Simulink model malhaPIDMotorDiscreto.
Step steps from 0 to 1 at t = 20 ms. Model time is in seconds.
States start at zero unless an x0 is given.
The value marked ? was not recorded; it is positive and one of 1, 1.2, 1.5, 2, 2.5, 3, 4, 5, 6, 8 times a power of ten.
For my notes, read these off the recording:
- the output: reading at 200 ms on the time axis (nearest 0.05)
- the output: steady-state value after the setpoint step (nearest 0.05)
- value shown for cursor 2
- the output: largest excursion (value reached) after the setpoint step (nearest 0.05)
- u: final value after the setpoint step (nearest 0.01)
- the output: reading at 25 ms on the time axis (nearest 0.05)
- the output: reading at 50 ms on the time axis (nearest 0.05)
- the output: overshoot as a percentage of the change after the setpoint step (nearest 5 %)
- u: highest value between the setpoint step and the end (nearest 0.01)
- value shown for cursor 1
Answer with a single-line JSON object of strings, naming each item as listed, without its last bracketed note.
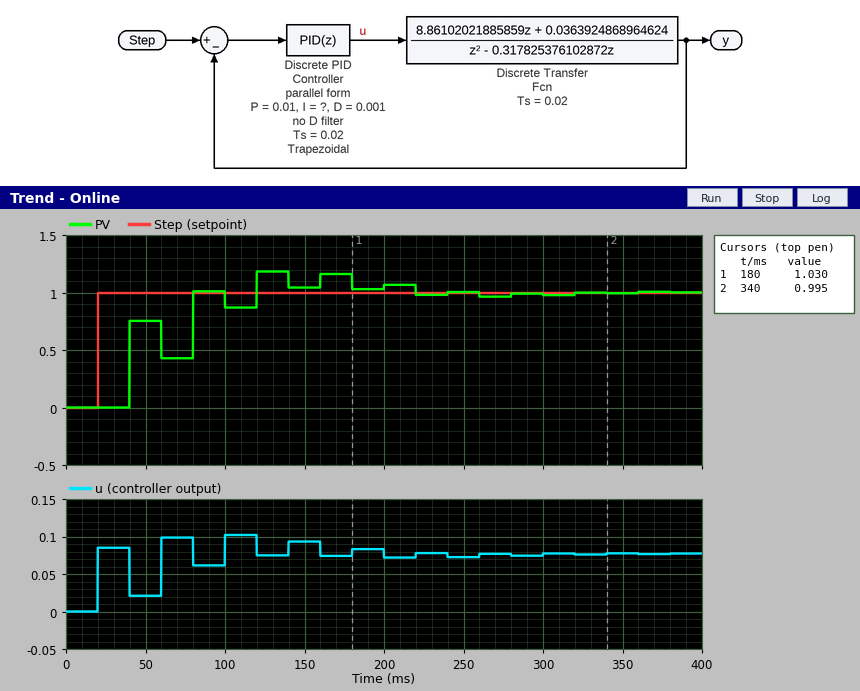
{"the output: reading at 200 ms on the time axis": "1.05", "the output: steady-state value after the setpoint step": "1.00", "value shown for cursor 2": "0.995", "the output: largest excursion (value reached) after the setpoint step": "1.20", "u: final value after the setpoint step": "0.08", "the output: reading at 25 ms on the time axis": "0.00", "the output: reading at 50 ms on the time axis": "0.75", "the output: overshoot as a percentage of the change after the setpoint step": "20 %", "u: highest value between the setpoint step and the end": "0.10", "value shown for cursor 1": "1.030"}
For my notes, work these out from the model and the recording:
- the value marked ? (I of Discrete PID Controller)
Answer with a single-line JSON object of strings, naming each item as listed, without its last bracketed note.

{"the value marked ?": "2.5"}
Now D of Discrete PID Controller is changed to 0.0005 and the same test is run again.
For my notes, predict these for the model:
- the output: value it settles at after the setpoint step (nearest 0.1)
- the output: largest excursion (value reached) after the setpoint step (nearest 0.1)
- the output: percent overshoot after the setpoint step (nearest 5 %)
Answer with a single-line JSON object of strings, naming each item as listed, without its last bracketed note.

{"the output: value it settles at after the setpoint step": "1.0", "the output: largest excursion (value reached) after the setpoint step": "1.1", "the output: percent overshoot after the setpoint step": "15 %"}
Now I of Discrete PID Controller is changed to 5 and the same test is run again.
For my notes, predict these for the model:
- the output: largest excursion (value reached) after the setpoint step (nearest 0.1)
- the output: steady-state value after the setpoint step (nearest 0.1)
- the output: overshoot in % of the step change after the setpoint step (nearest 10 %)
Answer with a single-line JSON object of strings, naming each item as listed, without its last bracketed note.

{"the output: largest excursion (value reached) after the setpoint step": "1.4", "the output: steady-state value after the setpoint step": "1.0", "the output: overshoot in % of the step change after the setpoint step": "40 %"}
